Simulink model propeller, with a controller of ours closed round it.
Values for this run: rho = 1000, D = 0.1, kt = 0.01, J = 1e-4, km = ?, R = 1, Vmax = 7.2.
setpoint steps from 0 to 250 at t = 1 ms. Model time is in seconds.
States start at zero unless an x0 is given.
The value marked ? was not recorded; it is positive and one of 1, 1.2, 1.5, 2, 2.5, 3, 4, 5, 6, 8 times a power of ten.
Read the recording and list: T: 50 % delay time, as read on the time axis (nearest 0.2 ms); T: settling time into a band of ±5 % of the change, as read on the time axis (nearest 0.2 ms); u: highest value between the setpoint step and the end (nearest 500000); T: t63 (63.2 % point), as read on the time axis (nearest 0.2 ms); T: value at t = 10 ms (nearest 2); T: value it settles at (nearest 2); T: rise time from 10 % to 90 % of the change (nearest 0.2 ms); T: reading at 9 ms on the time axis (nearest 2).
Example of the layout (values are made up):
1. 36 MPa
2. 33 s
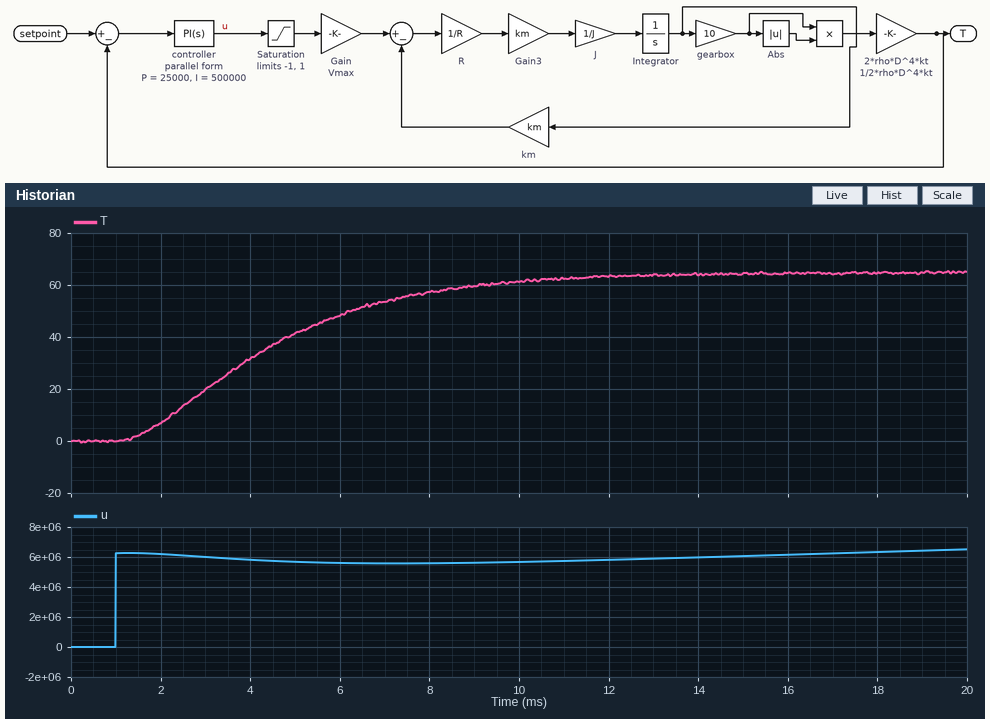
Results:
1. 4.0 ms
2. 10.2 ms
3. 6500000
4. 5.0 ms
5. 62
6. 64
7. 6.4 ms
8. 60
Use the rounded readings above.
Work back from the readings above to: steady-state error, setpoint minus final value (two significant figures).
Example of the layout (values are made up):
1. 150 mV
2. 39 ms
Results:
1. 190
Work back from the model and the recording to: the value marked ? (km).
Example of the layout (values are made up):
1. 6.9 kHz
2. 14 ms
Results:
1. 0.2
